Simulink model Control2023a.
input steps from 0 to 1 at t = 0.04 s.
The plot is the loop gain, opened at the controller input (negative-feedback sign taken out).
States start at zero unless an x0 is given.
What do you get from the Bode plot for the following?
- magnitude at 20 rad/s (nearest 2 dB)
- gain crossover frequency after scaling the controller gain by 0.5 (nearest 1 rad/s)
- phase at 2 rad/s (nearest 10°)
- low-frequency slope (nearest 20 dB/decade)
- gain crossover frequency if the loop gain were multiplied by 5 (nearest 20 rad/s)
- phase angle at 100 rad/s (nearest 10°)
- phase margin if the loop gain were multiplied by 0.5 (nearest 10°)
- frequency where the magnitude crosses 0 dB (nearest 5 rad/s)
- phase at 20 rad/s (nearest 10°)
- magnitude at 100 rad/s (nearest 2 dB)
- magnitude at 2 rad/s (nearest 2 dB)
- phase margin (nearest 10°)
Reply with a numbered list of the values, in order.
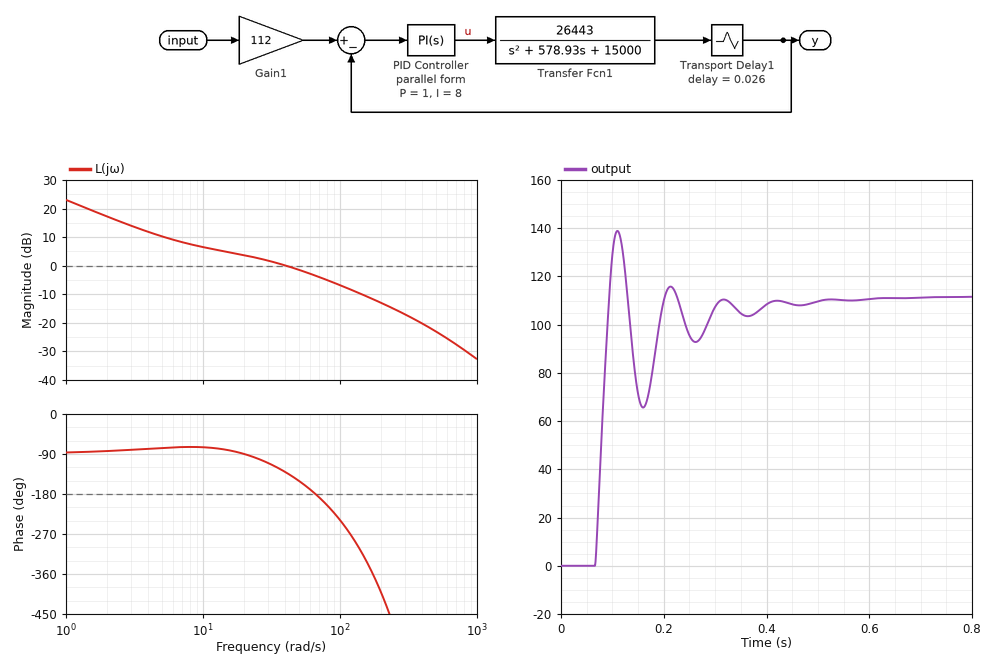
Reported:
1. 4 dB
2. 11 rad/s
3. -80°
4. -20 dB/decade
5. 220 rad/s
6. -240°
7. 100°
8. 40 rad/s
9. -90°
10. -6 dB
11. 18 dB
12. 50°
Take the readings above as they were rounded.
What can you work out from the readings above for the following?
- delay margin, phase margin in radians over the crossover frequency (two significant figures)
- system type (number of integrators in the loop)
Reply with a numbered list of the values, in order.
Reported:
1. 0.022 s
2. 1
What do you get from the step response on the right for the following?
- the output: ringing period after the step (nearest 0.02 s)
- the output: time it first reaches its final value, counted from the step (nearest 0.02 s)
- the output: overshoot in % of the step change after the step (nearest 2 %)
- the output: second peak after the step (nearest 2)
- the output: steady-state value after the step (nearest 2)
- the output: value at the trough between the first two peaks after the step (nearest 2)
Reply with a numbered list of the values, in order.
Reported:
1. 0.10 s
2. 0.06 s
3. 24 %
4. 116
5. 112
6. 66
